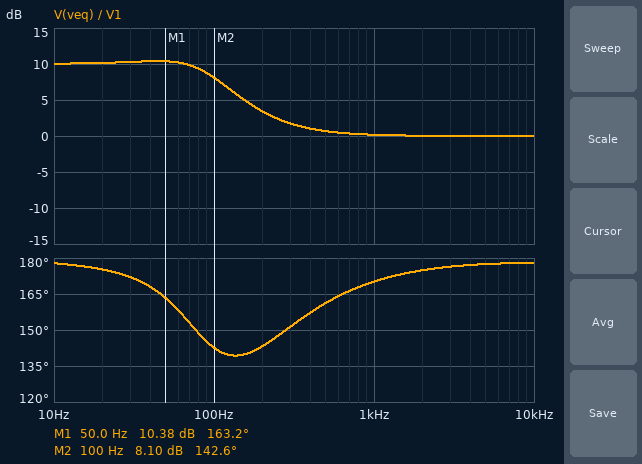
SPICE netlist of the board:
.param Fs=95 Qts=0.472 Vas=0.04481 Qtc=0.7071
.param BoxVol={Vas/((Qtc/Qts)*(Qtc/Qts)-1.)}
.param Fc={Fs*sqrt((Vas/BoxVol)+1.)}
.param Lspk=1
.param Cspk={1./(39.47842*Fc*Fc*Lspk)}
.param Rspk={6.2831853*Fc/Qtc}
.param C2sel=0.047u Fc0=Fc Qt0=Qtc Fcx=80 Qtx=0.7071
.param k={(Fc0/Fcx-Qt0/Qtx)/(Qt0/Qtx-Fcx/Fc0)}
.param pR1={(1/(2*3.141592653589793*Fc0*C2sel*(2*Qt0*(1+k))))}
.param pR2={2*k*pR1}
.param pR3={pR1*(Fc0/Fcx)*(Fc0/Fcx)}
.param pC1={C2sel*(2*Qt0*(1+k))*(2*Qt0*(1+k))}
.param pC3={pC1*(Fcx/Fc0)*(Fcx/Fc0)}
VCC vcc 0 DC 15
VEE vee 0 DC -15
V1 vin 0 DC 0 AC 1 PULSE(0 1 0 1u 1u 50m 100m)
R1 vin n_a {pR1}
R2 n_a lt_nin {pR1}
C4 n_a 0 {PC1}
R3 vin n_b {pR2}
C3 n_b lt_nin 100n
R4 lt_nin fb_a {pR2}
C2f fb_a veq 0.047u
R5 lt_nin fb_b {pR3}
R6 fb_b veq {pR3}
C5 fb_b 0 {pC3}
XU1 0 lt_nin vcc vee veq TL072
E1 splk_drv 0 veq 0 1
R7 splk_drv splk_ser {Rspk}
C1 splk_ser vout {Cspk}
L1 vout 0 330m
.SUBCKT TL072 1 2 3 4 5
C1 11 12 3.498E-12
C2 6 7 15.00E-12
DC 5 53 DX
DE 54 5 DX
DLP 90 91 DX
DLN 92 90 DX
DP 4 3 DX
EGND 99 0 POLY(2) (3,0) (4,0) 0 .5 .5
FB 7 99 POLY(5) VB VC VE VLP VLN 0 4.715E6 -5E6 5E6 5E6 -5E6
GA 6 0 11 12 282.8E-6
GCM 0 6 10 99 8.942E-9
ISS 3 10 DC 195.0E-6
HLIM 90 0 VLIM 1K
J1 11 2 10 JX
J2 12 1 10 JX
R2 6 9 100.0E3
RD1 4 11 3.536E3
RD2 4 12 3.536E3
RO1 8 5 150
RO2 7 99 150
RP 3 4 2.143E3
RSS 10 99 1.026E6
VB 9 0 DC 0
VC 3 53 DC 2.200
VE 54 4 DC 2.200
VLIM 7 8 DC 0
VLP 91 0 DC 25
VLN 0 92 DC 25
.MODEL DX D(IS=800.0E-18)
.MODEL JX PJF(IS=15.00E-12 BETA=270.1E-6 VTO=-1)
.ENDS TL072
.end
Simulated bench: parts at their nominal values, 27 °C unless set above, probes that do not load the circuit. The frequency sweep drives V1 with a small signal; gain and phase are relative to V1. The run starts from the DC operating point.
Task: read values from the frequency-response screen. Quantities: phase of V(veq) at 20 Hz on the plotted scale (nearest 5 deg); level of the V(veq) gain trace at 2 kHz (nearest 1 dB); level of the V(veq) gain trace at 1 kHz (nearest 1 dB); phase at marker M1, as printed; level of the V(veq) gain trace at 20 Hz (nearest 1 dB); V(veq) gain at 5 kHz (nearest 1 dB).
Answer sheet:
175 deg
0 dB
0 dB
163.2 deg
10 dB
0 dB
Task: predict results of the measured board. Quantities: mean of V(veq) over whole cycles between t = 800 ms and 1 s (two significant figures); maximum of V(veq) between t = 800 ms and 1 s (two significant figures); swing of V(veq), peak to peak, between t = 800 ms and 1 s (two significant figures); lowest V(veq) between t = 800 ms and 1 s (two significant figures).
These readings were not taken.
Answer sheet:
-1.6 V
220 mV
3.6 V
-3.4 V
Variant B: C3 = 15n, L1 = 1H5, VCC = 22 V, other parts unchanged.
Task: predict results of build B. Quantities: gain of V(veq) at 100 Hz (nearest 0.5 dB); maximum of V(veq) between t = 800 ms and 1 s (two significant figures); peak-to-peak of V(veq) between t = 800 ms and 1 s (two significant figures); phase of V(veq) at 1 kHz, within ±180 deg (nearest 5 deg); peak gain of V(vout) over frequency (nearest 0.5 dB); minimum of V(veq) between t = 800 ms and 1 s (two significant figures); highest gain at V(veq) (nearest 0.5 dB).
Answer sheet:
5.0 dB
150 mV
3.5 V
-170 deg
2.0 dB
-3.3 V
10.0 dB
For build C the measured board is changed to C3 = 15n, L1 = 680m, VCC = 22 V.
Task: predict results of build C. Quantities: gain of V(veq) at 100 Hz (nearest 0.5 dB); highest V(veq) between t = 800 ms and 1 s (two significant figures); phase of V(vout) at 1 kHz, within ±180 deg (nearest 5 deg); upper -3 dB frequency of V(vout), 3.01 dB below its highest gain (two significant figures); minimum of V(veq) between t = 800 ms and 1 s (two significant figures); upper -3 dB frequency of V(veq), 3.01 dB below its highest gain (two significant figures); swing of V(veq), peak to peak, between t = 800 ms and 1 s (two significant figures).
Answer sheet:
5.0 dB
150 mV
-150 deg
560 kHz
-3.3 V
83 Hz
3.5 V
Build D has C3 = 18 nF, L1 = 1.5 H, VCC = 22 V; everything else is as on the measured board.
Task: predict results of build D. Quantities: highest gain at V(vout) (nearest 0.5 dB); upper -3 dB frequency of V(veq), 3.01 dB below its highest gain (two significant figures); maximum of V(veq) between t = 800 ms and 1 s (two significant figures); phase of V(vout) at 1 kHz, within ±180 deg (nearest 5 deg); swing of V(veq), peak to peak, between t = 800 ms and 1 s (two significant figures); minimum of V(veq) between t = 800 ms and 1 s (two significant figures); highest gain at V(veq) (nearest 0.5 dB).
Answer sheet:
2.0 dB
82 Hz
150 mV
-165 deg
3.5 V
-3.3 V
10.0 dB
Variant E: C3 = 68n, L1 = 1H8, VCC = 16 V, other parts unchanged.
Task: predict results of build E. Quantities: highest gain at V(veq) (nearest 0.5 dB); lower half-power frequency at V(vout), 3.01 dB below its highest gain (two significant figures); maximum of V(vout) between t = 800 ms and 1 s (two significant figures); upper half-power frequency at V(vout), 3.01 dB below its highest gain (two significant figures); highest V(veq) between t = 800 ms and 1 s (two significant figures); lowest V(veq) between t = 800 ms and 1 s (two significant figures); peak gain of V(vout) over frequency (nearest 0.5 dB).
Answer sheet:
10.0 dB
72 Hz
1.0 V
210 Hz
120 mV
-3.3 V
6.0 dB
